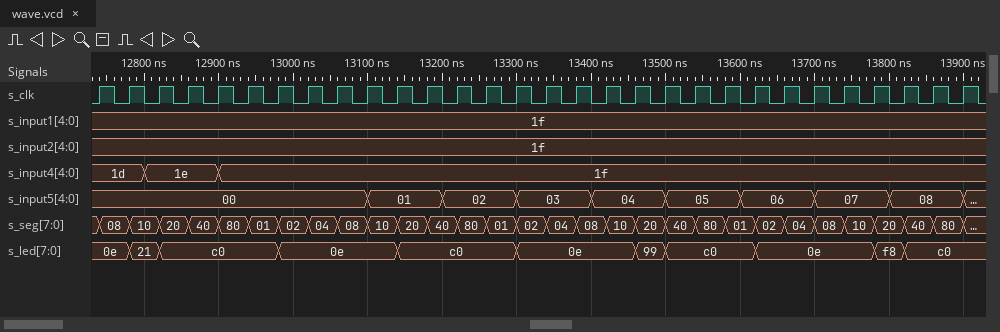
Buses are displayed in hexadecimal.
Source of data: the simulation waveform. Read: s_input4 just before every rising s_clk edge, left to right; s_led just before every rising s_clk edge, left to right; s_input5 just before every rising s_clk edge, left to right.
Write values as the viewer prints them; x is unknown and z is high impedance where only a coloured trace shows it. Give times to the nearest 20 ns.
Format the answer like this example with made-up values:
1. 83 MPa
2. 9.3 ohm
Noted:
1. 1d, 1d, 1e, 1e, 1e, 1f, 1f, 1f, 1f, 1f, 1f, 1f, 1f, 1f, 1f, 1f, 1f, 1f, 1f, 1f, 1f, 1f, 1f, 1f, 1f, 1f, 1f, 1f, 1f, 1f
2. 0e, 0e, 21, c0, c0, c0, c0, 0e, 0e, 0e, 0e, c0, c0, c0, c0, 0e, 0e, 0e, 0e, 99, c0, c0, c0, 0e, 0e, 0e, 0e, f8, c0, c0
3. 00, 00, 00, 00, 00, 00, 00, 00, 00, 00, 01, 01, 02, 02, 02, 03, 03, 04, 04, 04, 05, 05, 06, 06, 06, 07, 07, 08, 08, 08
